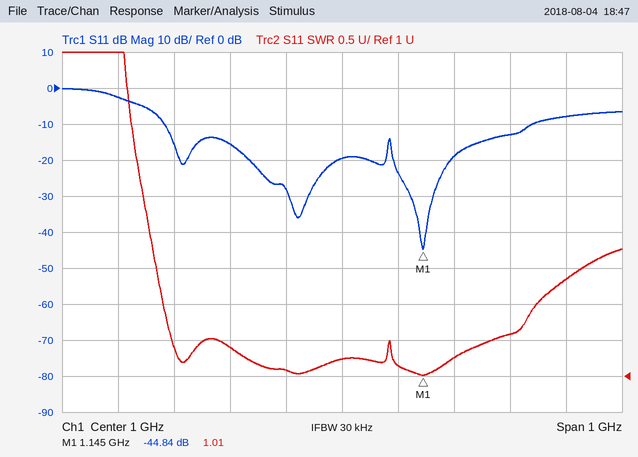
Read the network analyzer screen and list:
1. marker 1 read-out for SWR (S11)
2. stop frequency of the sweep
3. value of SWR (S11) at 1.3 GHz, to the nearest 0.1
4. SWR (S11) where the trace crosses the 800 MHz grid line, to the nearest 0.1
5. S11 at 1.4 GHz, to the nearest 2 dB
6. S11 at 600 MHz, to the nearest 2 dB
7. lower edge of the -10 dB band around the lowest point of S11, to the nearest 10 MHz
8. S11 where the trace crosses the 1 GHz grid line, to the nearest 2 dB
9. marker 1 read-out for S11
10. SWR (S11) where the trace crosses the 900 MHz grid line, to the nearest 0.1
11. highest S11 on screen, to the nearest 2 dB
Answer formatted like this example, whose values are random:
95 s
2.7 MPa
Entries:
1.01
1.5 GHz
1.6
1.4
-8 dB
-2 dB
680 MHz
-20 dB
-44.84 dB
1.1
0 dB
